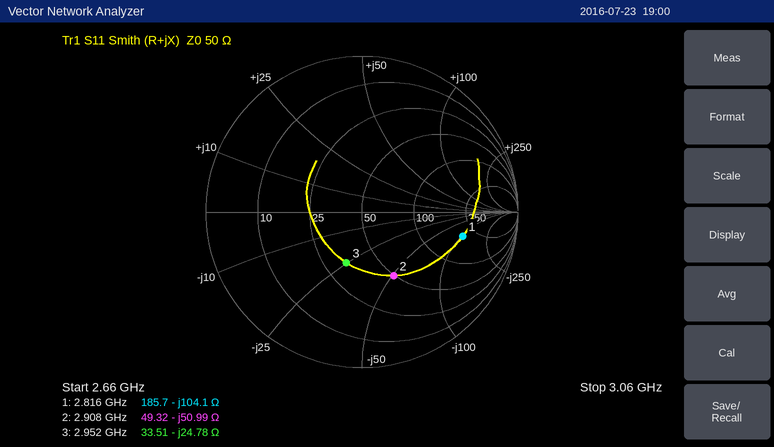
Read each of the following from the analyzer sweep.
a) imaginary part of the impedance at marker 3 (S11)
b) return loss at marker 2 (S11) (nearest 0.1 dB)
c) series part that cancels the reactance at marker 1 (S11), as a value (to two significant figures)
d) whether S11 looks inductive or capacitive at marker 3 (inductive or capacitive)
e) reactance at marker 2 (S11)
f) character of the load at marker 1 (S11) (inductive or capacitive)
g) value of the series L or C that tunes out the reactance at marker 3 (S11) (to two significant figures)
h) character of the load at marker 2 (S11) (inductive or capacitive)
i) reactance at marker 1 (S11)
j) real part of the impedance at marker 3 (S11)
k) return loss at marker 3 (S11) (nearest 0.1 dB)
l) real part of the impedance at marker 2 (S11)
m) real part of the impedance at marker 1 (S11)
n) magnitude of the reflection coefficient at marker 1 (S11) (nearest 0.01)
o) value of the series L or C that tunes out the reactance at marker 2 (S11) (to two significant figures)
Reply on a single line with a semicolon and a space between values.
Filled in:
-24.78 Ω; 6.8 dB; 5.9 nH; capacitive; -50.99 Ω; capacitive; 1.3 nH; capacitive; -104.1 Ω; 33.51 Ω; 9.3 dB; 49.32 Ω; 185.7 Ω; 0.66; 2.8 nH
